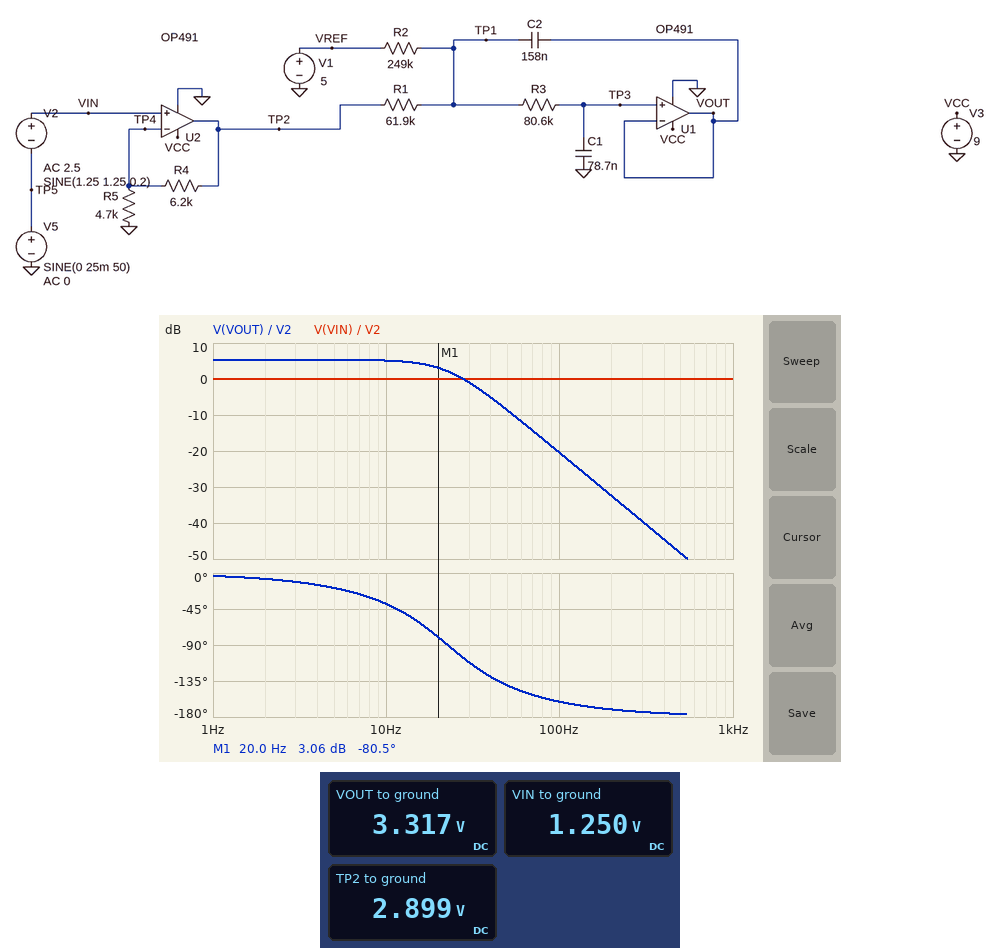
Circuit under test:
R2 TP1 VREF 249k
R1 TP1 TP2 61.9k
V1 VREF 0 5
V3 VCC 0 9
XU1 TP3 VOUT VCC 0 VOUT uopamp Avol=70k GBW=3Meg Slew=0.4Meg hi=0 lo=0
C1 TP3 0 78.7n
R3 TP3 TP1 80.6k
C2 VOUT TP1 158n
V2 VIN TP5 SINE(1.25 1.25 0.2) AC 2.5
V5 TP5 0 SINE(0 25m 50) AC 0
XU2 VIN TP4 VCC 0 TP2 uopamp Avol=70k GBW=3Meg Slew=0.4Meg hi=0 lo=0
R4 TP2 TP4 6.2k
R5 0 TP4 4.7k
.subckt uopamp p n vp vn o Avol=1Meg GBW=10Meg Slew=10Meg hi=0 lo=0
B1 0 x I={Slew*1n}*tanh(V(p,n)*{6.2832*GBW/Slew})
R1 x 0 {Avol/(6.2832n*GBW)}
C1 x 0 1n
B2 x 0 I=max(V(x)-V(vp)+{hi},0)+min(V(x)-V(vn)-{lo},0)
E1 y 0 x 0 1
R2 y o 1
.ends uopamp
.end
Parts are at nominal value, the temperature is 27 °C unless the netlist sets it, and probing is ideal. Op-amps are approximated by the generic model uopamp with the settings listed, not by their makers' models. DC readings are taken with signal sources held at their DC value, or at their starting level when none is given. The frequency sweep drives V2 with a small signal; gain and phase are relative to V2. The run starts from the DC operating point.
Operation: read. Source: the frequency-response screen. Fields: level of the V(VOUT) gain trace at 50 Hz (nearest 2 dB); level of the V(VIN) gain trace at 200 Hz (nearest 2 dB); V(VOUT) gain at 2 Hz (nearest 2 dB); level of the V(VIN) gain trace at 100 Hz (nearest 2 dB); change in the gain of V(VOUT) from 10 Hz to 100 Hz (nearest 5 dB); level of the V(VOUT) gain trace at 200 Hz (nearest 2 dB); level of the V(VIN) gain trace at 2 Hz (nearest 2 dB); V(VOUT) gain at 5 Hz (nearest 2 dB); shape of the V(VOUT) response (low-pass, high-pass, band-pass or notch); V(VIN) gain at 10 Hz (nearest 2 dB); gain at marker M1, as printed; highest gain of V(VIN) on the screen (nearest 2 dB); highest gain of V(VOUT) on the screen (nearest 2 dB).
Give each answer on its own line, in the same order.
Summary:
-8 dB
0 dB
6 dB
0 dB
-25 dB
-32 dB
0 dB
6 dB
low-pass
0 dB
3.06 dB
0 dB
6 dB
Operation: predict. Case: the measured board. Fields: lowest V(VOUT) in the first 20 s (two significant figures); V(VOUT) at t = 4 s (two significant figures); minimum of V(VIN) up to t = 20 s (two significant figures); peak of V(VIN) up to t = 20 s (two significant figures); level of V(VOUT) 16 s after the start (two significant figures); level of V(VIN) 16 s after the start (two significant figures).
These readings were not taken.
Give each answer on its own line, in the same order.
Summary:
1.0 V
1.1 V
-25 mV
2.5 V
5.5 V
2.4 V
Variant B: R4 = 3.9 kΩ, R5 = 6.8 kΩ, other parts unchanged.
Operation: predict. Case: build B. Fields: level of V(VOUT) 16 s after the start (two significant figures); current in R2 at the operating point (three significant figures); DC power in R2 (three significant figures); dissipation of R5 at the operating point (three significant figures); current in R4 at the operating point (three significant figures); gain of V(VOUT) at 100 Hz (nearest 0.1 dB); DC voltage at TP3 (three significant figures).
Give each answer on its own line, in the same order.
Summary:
4.1 V
9.76 µA
23.7 µW
230 µW
184 µA
-23.9 dB
2.57 V
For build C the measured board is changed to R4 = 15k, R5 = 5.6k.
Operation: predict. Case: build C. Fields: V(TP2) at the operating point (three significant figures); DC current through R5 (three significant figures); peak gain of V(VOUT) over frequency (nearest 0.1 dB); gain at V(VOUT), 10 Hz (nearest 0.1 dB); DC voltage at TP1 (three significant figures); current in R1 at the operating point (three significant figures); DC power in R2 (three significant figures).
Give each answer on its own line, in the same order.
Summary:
4.60 V
223 µA
9.4 dB
9.1 dB
4.68 V
1.29 µA
416 nW
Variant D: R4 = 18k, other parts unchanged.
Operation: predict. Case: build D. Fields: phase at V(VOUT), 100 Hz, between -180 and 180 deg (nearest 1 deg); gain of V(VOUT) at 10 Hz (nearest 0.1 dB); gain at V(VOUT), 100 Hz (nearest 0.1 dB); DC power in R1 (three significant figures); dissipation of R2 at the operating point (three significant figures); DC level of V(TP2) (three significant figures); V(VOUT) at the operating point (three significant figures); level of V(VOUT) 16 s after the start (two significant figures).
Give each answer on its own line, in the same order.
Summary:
-161 deg
11.5 dB
-14.1 dB
688 nW
2.77 µW
6.04 V
5.83 V
8.2 V
